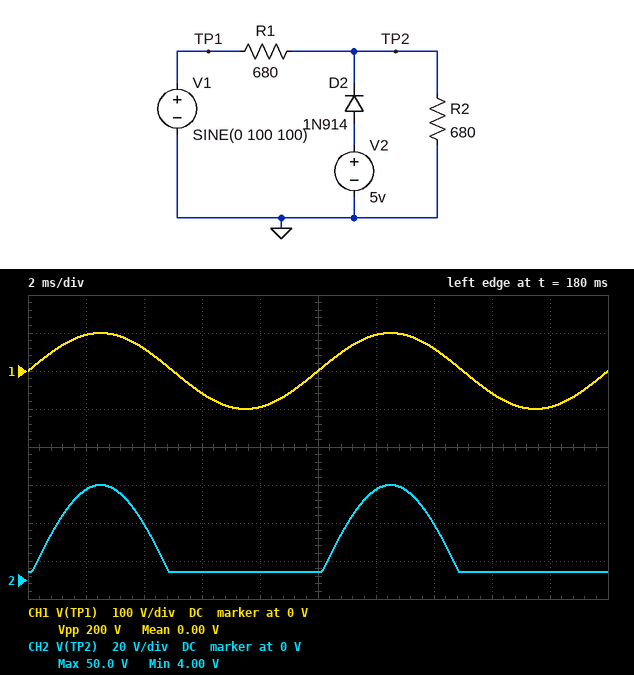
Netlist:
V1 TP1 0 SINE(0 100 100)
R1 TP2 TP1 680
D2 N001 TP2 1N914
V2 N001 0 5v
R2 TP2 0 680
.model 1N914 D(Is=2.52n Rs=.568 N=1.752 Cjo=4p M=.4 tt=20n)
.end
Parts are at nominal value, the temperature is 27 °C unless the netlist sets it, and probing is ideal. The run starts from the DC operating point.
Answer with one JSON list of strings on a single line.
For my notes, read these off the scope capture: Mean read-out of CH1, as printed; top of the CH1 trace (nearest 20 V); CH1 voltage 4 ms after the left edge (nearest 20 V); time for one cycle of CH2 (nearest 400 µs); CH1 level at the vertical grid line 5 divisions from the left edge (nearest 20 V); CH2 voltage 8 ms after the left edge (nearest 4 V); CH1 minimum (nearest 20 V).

["0.00 V", "100 V", "60 V", "10.0 ms", "0 V", "4 V", "-100 V"]
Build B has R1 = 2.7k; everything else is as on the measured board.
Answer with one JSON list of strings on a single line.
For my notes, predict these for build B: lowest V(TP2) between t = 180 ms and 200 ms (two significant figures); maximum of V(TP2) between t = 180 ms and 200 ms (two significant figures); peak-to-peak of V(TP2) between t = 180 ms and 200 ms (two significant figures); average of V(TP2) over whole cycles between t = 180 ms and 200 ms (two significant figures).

["4.2 V", "20 V", "16 V", "8.7 V"]
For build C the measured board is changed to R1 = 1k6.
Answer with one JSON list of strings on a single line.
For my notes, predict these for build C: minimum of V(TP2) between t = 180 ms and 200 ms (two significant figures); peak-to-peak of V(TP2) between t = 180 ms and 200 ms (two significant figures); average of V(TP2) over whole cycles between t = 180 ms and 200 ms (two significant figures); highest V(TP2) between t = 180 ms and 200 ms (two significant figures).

["4.2 V", "26 V", "12 V", "30 V"]
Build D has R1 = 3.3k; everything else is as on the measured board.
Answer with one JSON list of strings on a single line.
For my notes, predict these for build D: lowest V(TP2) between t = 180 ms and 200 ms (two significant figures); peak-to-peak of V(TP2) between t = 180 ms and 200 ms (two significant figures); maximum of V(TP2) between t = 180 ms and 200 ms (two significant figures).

["4.2 V", "13 V", "17 V"]
